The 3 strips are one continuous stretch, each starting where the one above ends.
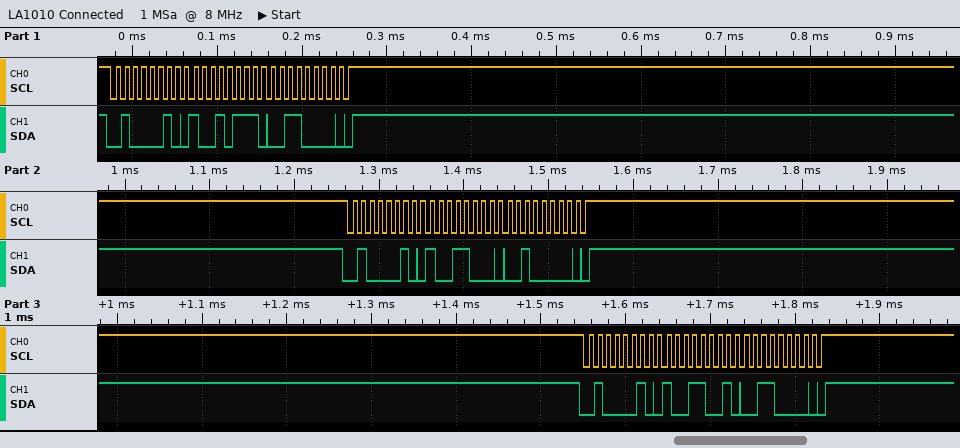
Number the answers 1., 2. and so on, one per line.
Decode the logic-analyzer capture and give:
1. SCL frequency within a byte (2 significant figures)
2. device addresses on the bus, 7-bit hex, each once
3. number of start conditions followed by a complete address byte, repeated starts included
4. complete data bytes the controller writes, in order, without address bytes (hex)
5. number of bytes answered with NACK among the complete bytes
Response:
1. 100 kHz
2. 0x21
3. 3
4. 97 30 98 20 99 30
5. 0
